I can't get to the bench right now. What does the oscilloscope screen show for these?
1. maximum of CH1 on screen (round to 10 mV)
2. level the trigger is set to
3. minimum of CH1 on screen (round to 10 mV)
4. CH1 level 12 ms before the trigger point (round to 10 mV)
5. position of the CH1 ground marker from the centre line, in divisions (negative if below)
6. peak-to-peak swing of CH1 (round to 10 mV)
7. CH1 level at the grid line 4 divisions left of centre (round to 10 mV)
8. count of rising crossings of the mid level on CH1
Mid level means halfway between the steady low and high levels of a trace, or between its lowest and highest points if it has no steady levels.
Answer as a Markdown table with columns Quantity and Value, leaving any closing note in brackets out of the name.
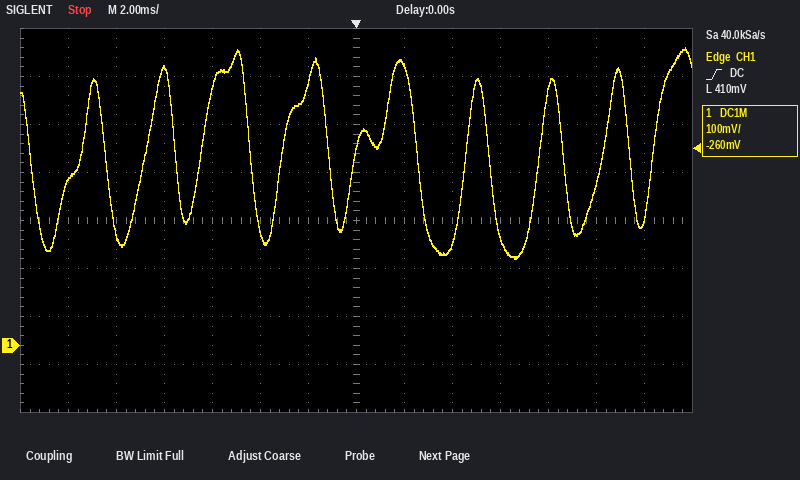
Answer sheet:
| Quantity | Value |
|---|---|
| maximum of CH1 on screen | 620 mV |
| level the trigger is set to | 410 mV |
| minimum of CH1 on screen | 180 mV |
| CH1 level 12 ms before the trigger point | 340 mV |
| position of the CH1 ground marker from the centre line, in divisions | -2.6 div |
| peak-to-peak swing of CH1 | 440 mV |
| CH1 level at the grid line 4 divisions left of centre | 580 mV |
| count of rising crossings of the mid level on CH1 | 9 |
